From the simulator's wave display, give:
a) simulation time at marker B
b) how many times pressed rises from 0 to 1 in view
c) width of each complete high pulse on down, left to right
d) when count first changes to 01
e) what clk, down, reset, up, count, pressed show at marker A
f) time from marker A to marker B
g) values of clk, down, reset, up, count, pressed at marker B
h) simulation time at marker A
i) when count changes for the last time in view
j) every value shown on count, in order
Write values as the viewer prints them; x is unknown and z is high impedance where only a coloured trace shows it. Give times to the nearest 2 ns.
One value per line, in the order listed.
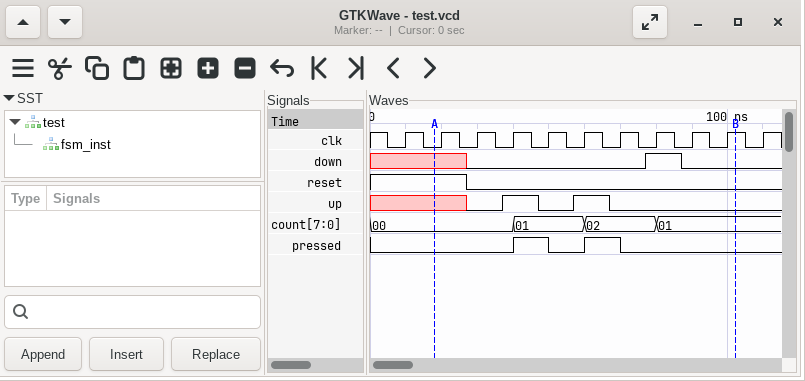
102 ns
2
10 ns
40 ns
clk=0, down=x, reset=1, up=x, count=00, pressed=0
84 ns
clk=1, down=0, reset=0, up=0, count=01, pressed=0
18 ns
80 ns
00, 01, 02, 01
